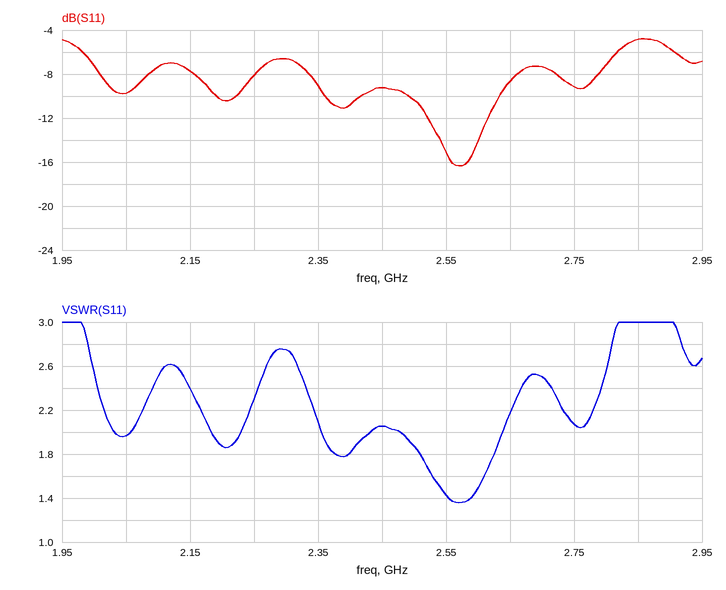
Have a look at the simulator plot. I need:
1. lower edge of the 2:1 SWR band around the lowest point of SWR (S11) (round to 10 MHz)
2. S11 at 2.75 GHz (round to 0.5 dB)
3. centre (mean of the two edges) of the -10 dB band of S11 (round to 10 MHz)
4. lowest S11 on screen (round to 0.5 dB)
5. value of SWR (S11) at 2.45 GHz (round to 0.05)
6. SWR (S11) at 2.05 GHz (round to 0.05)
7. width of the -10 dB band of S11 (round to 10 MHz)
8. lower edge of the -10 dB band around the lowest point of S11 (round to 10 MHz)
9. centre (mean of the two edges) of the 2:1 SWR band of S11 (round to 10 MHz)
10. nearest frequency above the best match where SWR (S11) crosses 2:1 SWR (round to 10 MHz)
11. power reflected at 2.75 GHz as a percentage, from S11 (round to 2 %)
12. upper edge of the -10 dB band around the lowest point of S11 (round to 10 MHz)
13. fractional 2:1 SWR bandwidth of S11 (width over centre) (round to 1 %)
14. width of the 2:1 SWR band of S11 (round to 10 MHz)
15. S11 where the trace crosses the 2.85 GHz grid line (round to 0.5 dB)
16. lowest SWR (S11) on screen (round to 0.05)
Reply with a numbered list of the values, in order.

1. 2.48 GHz
2. -9.0 dB
3. 2.56 GHz
4. -16.5 dB
5. 2.05
6. 1.95
7. 140 MHz
8. 2.49 GHz
9. 2.56 GHz
10. 2.64 GHz
11. 12 %
12. 2.63 GHz
13. 6 %
14. 160 MHz
15. -5.0 dB
16. 1.35
